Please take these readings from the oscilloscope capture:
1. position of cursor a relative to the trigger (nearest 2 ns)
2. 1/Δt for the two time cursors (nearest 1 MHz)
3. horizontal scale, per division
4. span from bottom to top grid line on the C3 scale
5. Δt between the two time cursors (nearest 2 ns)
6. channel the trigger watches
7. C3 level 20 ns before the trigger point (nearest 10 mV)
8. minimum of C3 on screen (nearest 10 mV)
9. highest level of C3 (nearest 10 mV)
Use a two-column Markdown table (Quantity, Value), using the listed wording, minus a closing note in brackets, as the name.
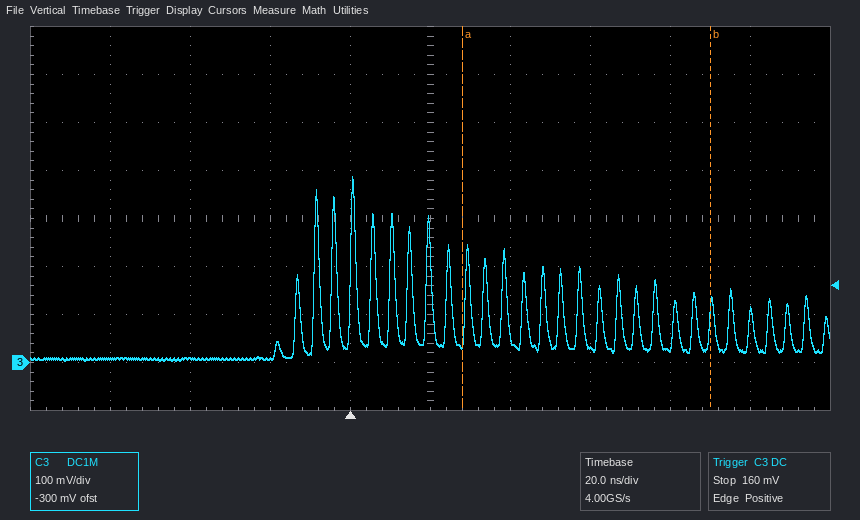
| Quantity | Value |
|---|---|
| position of cursor a relative to the trigger | +28 ns |
| 1/Δt for the two time cursors | 16 MHz |
| horizontal scale, per division | 20 ns |
| span from bottom to top grid line on the C3 scale | 800 mV |
| Δt between the two time cursors | 62 ns |
| channel the trigger watches | C3 |
| C3 level 20 ns before the trigger point | 10 mV |
| minimum of C3 on screen | 0 mV |
| highest level of C3 | 390 mV |
